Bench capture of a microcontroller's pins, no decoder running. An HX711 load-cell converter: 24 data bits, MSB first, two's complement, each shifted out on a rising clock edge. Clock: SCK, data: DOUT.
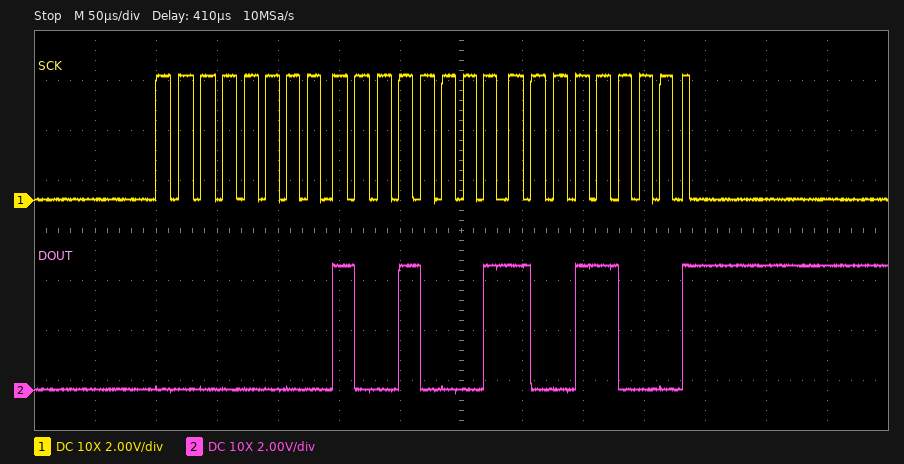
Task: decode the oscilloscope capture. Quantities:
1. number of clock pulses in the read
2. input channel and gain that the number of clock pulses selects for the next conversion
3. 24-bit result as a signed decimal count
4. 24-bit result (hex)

25
channel A, gain 128
37272
0x009198
